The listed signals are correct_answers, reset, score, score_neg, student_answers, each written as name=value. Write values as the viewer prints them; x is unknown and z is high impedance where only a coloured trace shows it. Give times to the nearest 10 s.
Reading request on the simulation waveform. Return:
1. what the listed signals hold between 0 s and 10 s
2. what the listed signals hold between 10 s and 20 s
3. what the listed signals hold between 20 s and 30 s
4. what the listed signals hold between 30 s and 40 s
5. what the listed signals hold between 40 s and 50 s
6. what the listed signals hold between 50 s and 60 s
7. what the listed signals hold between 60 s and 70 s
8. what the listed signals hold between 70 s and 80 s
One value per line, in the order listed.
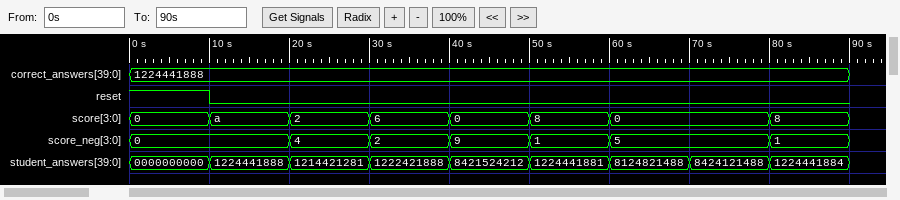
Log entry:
correct_answers=1224441888, reset=1, score=0, score_neg=0, student_answers=0000000000
correct_answers=1224441888, reset=0, score=a, score_neg=0, student_answers=1224441888
correct_answers=1224441888, reset=0, score=2, score_neg=4, student_answers=1214421281
correct_answers=1224441888, reset=0, score=6, score_neg=2, student_answers=1222421888
correct_answers=1224441888, reset=0, score=0, score_neg=9, student_answers=8421524212
correct_answers=1224441888, reset=0, score=8, score_neg=1, student_answers=1224441881
correct_answers=1224441888, reset=0, score=0, score_neg=5, student_answers=8124821488
correct_answers=1224441888, reset=0, score=0, score_neg=5, student_answers=8424121488
